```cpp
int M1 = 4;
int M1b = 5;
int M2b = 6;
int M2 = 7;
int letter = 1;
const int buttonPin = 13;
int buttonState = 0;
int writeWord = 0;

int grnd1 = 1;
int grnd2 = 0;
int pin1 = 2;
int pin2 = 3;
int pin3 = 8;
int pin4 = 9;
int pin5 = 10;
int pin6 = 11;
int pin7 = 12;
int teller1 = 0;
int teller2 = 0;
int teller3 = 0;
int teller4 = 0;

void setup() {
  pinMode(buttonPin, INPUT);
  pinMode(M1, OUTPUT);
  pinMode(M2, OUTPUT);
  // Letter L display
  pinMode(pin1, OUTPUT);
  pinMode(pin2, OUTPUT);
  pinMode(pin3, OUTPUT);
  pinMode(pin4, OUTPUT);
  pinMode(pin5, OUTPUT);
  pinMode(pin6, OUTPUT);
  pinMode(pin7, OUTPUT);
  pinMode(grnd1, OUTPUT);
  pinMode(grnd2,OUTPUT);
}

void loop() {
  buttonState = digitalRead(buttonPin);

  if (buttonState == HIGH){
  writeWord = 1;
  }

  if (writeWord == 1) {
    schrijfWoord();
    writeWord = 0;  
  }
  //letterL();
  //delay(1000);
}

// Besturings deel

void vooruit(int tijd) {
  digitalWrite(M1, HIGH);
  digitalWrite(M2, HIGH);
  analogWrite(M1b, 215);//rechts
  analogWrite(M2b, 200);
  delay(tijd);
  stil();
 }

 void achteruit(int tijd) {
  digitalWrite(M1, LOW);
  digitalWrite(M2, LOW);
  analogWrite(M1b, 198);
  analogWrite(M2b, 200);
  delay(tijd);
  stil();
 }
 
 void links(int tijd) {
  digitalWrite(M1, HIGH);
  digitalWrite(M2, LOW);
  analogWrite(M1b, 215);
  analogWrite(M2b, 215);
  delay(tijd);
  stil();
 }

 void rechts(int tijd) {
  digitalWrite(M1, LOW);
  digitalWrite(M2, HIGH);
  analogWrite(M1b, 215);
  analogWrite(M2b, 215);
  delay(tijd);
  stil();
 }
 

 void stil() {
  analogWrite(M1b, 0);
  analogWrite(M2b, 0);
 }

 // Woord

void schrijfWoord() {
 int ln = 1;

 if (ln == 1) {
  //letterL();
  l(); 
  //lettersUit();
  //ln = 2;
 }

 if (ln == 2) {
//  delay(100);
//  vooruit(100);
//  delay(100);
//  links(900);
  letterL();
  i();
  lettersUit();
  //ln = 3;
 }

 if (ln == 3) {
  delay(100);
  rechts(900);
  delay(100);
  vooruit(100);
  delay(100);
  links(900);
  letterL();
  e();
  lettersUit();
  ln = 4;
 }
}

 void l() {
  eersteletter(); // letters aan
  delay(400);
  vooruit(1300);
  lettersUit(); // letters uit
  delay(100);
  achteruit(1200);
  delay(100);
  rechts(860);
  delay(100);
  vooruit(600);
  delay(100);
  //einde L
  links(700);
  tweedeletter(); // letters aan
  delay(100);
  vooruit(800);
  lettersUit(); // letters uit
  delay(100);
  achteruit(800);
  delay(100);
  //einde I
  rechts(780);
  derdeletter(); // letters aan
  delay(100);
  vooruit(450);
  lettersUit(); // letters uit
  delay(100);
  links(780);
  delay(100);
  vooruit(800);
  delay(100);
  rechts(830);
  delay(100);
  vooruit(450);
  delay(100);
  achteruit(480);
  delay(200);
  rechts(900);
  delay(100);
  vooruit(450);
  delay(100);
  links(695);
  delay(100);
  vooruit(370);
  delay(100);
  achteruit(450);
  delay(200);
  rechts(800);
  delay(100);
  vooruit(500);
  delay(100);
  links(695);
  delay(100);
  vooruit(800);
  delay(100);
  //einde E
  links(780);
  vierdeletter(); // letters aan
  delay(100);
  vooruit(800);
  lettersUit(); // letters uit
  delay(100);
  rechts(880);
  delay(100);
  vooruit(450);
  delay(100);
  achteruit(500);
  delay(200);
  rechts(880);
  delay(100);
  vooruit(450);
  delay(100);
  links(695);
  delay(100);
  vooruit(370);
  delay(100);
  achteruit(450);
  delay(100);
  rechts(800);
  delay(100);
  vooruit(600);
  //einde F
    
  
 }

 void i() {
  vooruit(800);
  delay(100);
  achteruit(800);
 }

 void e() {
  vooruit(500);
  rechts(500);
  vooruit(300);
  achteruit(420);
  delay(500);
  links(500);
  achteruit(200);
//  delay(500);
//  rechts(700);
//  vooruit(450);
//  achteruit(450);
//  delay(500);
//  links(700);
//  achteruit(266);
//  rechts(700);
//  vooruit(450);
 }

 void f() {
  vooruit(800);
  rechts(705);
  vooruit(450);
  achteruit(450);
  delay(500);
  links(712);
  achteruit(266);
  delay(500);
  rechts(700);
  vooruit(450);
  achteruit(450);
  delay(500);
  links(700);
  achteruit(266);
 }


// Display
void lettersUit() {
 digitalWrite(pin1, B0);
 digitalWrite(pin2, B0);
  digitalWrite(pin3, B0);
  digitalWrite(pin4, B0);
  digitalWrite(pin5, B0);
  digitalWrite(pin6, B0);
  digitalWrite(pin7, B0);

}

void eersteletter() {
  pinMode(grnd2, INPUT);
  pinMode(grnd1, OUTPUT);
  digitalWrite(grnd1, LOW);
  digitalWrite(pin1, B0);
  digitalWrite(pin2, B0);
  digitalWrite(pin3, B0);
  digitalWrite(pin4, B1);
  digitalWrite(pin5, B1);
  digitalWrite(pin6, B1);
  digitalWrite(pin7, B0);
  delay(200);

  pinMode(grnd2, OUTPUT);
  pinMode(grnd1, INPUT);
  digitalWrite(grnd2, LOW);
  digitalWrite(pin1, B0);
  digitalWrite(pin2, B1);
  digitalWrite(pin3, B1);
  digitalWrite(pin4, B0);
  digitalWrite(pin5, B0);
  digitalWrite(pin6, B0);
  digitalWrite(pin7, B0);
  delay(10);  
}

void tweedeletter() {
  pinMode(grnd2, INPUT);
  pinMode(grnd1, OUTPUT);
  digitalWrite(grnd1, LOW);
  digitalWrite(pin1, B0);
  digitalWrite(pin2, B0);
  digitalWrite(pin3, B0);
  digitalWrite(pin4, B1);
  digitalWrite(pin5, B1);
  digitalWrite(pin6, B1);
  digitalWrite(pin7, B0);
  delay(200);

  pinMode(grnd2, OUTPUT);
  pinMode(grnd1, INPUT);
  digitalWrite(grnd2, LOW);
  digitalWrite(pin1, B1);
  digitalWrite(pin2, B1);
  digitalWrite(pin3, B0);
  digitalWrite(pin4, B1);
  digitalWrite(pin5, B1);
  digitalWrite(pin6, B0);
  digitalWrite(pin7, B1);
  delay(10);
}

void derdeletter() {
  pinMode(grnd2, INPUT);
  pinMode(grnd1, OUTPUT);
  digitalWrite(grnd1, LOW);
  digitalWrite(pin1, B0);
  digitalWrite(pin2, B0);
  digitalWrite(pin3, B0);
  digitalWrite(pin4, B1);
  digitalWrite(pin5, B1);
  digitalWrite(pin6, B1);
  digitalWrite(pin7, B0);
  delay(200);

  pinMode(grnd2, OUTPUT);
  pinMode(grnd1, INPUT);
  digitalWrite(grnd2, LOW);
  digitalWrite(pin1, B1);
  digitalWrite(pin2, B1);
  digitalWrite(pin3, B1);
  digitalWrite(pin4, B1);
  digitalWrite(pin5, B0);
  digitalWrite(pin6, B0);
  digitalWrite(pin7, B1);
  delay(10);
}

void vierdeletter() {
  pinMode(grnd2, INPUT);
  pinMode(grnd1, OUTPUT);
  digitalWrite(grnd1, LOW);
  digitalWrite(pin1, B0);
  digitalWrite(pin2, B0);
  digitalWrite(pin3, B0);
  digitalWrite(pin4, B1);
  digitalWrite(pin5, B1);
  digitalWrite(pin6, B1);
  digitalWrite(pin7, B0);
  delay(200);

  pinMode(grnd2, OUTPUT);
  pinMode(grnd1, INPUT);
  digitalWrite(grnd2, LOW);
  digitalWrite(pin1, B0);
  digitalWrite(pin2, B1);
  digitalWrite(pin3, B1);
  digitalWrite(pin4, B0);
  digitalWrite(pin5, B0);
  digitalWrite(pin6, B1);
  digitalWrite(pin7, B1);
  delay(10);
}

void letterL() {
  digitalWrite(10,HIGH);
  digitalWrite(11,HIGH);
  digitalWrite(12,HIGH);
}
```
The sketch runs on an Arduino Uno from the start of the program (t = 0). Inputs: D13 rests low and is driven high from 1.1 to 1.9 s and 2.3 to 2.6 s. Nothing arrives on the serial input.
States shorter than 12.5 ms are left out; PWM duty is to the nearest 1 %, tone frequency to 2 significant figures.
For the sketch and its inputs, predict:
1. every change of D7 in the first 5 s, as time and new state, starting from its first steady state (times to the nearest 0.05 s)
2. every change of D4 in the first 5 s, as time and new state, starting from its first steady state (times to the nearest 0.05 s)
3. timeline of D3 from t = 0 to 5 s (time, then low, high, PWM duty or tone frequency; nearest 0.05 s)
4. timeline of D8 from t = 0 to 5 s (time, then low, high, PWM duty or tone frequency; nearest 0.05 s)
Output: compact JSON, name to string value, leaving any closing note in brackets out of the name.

{"every change of D7 in the first 5 s, as time and new state, starting from its first steady state": "0 s low; 1.7 s high; 3.1 s low; 4.4 s high", "every change of D4 in the first 5 s, as time and new state, starting from its first steady state": "0 s low; 1.7 s high; 3.1 s low", "timeline of D3 from t = 0 to 5 s": "0 s low; 1.3 s high; 3 s low", "timeline of D8 from t = 0 to 5 s": "0 s low; 1.3 s high; 3 s low"}
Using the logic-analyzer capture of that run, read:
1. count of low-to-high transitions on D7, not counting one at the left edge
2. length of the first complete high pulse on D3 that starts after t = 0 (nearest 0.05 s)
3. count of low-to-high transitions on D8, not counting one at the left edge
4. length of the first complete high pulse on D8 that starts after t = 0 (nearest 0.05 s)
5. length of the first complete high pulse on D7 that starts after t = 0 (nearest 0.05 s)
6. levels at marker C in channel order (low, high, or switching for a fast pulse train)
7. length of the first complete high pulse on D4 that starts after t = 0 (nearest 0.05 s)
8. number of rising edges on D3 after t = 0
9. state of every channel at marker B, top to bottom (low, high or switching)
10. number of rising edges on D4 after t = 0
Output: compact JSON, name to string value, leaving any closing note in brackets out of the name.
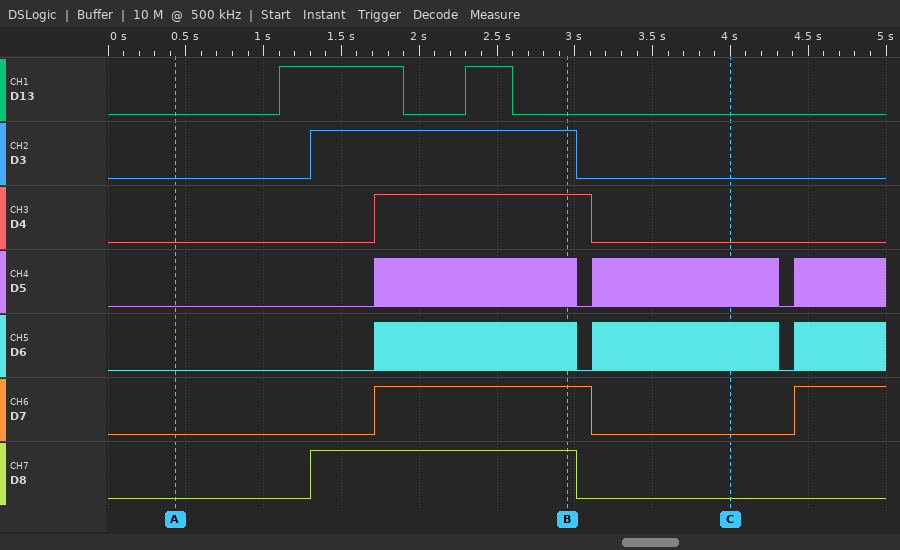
{"count of low-to-high transitions on D7, not counting one at the left edge": "2", "length of the first complete high pulse on D3 that starts after t = 0": "1.70 s", "count of low-to-high transitions on D8, not counting one at the left edge": "1", "length of the first complete high pulse on D8 that starts after t = 0": "1.70 s", "length of the first complete high pulse on D7 that starts after t = 0": "1.40 s", "levels at marker C in channel order": "D13 low, D3 low, D4 low, D5 switching, D6 switching, D7 low, D8 low", "length of the first complete high pulse on D4 that starts after t = 0": "1.40 s", "number of rising edges on D3 after t = 0": "1", "state of every channel at marker B, top to bottom": "D13 low, D3 high, D4 high, D5 switching, D6 switching, D7 high, D8 high", "number of rising edges on D4 after t = 0": "1"}
